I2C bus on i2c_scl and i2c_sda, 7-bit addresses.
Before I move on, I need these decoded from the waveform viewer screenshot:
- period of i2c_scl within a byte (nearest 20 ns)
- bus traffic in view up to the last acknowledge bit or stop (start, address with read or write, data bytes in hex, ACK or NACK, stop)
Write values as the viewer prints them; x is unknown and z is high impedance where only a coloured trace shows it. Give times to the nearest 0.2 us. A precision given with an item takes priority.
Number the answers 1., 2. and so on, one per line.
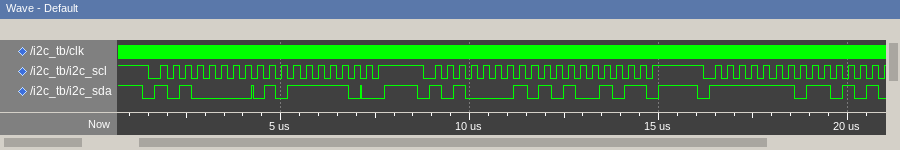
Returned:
1. 320 ns
2. start, address 50 write ACK, BE ACK, stop, start, address 50 read ACK, A5 NACK, stop, start, address 7F write NACK
